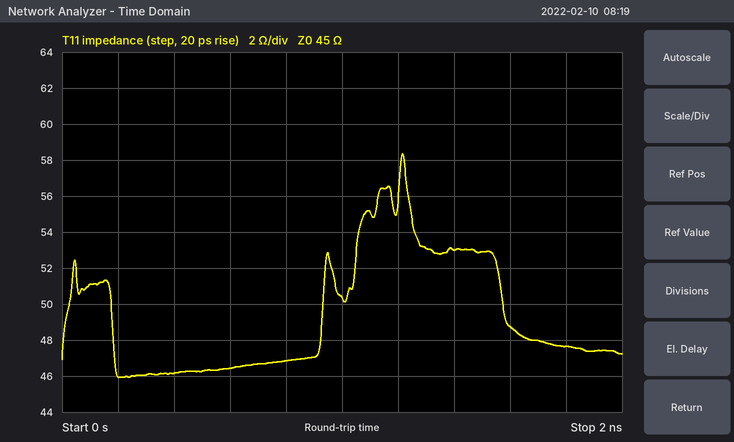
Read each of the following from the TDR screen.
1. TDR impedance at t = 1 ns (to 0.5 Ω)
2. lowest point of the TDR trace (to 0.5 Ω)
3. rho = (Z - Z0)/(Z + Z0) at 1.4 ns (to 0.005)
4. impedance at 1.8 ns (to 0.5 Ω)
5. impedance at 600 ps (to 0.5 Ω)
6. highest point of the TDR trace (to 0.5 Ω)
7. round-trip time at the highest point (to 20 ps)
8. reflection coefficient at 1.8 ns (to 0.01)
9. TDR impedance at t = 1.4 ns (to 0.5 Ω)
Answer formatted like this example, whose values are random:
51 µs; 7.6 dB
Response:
50.5 Ω; 46.0 Ω; +0.080; 47.5 Ω; 46.5 Ω; 58.5 Ω; 1.22 ns; +0.03; 53.0 Ω
